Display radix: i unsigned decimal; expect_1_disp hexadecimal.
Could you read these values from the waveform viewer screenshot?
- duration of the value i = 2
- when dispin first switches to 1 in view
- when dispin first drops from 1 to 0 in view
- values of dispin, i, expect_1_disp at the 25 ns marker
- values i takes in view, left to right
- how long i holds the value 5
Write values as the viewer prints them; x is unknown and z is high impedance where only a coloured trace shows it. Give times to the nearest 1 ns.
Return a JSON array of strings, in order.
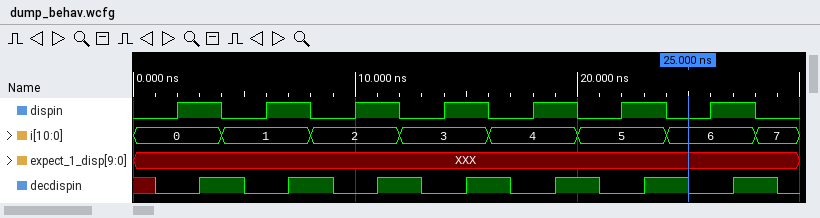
["4 ns", "2 ns", "4 ns", "dispin=0, i=6, expect_1_disp=XXX", "0, 1, 2, 3, 4, 5, 6, 7", "4 ns"]
